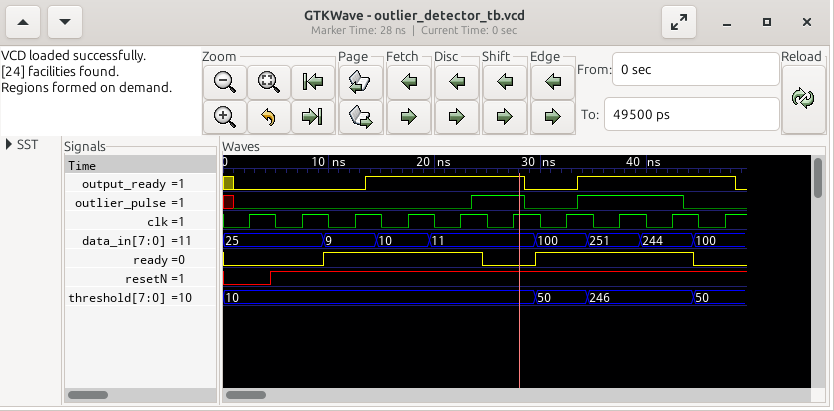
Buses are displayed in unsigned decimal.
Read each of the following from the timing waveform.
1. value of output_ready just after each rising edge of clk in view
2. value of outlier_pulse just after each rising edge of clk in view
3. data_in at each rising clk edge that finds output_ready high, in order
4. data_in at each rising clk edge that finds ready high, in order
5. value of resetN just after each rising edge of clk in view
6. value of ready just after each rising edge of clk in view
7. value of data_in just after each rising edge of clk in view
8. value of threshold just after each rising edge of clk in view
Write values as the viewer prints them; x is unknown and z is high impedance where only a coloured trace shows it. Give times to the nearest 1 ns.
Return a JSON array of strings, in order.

["0 0 0 1 1 1 0 1 1 1", "0 0 0 0 0 1 0 1 1 0", "10, 11, 11, 251, 244, 100", "9, 10, 11, 100, 251, 244", "0 1 1 1 1 1 1 1 1 1", "0 0 1 1 1 0 1 1 1 0", "25, 25, 9, 10, 11, 11, 100, 251, 244, 100", "10, 10, 10, 10, 10, 10, 50, 246, 246, 50"]
